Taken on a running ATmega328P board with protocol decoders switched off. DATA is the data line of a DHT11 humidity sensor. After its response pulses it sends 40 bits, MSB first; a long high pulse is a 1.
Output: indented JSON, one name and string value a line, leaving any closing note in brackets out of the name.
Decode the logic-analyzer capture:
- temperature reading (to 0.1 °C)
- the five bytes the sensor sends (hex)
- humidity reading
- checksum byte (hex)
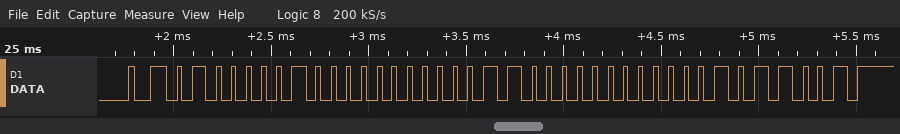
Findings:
{
  "temperature reading": "24.0 °C",
  "the five bytes the sensor sends": "41 00 18 00 59",
  "humidity reading": "65 %",
  "checksum byte": "0x59"
}
